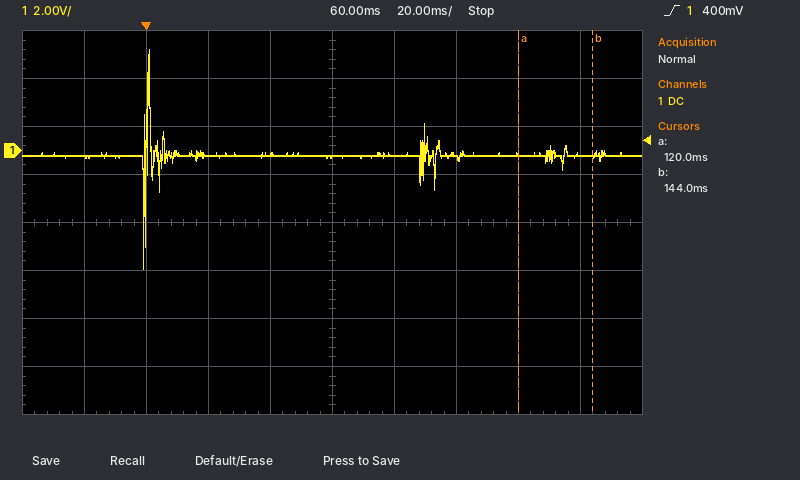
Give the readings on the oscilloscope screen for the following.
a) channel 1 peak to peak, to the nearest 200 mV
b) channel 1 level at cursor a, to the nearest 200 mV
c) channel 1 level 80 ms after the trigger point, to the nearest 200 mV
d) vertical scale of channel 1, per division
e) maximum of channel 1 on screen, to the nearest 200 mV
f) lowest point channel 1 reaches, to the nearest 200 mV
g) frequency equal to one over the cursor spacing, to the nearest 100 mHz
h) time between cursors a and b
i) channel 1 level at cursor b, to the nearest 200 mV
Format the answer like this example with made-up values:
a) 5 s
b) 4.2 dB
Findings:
a) 9.2 V
b) -200 mV
c) -200 mV
d) 2 V
e) 4.2 V
f) -5.0 V
g) 41.7 Hz
h) 24 ms
i) -200 mV
